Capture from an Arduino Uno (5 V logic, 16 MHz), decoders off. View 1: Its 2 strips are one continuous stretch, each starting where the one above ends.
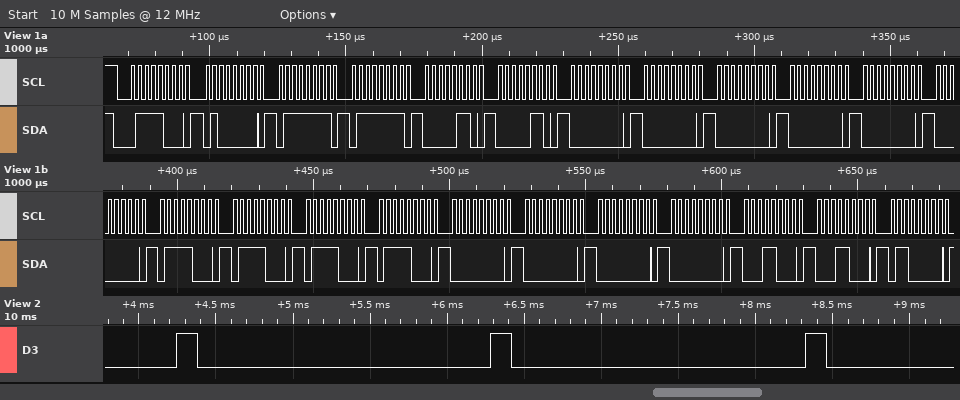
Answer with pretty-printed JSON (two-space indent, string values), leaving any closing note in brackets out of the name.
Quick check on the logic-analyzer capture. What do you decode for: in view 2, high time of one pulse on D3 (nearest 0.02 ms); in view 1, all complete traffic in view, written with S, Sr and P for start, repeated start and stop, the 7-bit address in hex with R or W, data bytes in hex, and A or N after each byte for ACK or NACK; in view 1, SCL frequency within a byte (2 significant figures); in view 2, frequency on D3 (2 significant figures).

{
  "in view 2, high time of one pulse on D3": "0.14 ms",
  "in view 1, all complete traffic in view, written with S, Sr and P for start, repeated start and stop, the 7-bit address in hex with R or W, data bytes in hex, and A or N after each byte for ACK or NACK": "S 3CW A 40 A 7F A 7F A 06 A 06 A 00 A 00 A 00 A 00 A 00 A 00 A 78 A 78 A 78 A 78 A 00 A 00 A 00 A 00 A 18 A 18 A 60 A",
  "in view 1, SCL frequency within a byte": "400 kHz",
  "in view 2, frequency on D3": "490 Hz"
}
